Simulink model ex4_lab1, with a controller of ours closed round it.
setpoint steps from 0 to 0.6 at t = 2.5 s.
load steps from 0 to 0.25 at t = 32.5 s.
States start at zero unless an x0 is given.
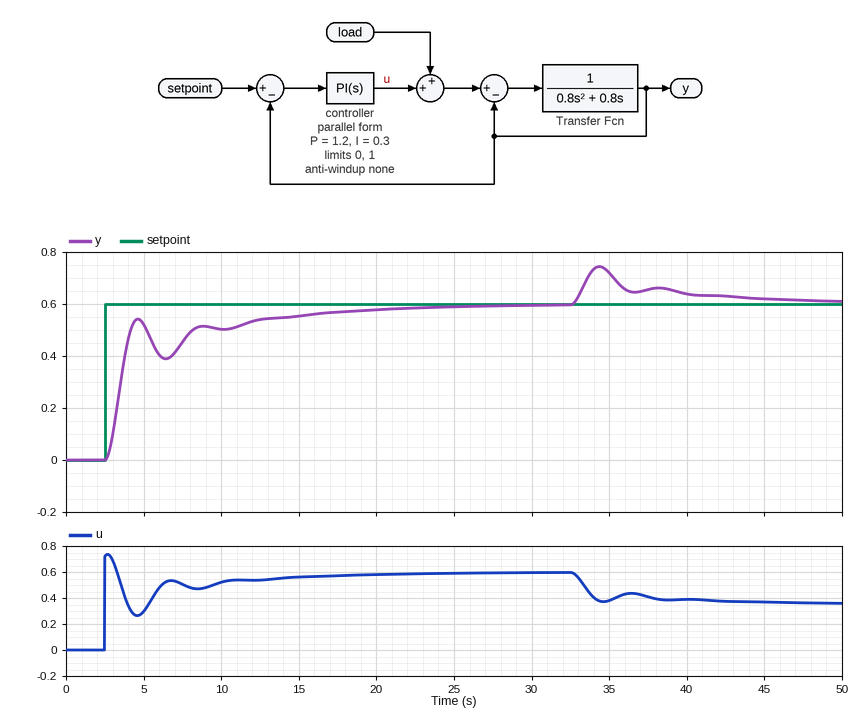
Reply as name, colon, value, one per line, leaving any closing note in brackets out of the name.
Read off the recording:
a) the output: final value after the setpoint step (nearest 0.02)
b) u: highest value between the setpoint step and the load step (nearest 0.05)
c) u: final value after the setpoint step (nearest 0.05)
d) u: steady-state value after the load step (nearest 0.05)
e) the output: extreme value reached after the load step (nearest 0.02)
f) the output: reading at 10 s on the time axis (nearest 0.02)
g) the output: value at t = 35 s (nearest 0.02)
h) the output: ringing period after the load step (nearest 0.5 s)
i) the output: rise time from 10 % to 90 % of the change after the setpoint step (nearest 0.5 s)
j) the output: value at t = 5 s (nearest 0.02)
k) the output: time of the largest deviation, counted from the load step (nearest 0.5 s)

the output: final value after the setpoint step: 0.60
u: highest value between the setpoint step and the load step: 0.75
u: final value after the setpoint step: 0.60
u: steady-state value after the load step: 0.35
the output: extreme value reached after the load step: 0.74
the output: reading at 10 s on the time axis: 0.50
the output: value at t = 35 s: 0.72
the output: ringing period after the load step: 4.0 s
the output: rise time from 10 % to 90 % of the change after the setpoint step: 1.5 s
the output: value at t = 5 s: 0.52
the output: time of the largest deviation, counted from the load step: 2.0 s
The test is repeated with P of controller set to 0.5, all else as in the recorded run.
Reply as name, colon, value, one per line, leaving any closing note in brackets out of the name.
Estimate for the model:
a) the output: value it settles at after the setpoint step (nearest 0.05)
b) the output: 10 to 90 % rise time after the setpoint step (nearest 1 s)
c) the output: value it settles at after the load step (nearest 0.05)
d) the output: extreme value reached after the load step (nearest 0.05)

the output: value it settles at after the setpoint step: 0.60
the output: 10 to 90 % rise time after the setpoint step: 7 s
the output: value it settles at after the load step: 0.60
the output: extreme value reached after the load step: 0.80
